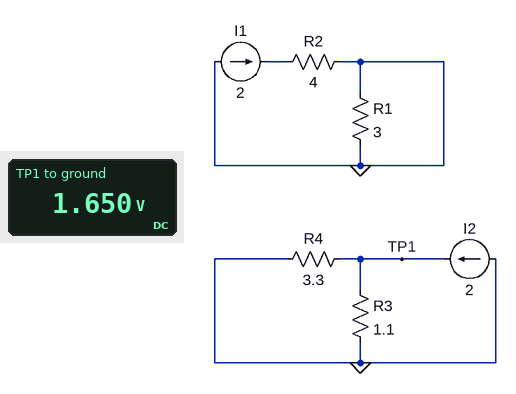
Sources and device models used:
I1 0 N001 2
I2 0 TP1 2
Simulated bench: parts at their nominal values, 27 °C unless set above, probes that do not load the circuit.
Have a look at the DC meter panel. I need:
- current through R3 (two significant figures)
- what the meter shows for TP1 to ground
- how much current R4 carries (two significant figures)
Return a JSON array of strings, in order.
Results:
["1.5 A", "1.650 V", "500 mA"]
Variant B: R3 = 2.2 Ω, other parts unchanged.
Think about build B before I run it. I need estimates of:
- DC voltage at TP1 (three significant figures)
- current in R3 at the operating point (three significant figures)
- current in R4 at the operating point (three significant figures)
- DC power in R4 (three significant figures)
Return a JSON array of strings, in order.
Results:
["2.64 V", "1.20 A", "800 mA", "2.11 W"]
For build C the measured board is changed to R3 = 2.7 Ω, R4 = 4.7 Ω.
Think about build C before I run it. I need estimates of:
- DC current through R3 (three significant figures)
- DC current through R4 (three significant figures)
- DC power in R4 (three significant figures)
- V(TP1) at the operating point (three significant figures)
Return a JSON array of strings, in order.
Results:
["1.27 A", "730 mA", "2.50 W", "3.43 V"]
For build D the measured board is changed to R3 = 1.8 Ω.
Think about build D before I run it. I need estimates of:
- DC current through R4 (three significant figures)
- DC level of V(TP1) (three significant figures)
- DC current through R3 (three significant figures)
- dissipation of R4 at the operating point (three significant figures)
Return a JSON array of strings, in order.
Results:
["706 mA", "2.33 V", "1.29 A", "1.64 W"]
